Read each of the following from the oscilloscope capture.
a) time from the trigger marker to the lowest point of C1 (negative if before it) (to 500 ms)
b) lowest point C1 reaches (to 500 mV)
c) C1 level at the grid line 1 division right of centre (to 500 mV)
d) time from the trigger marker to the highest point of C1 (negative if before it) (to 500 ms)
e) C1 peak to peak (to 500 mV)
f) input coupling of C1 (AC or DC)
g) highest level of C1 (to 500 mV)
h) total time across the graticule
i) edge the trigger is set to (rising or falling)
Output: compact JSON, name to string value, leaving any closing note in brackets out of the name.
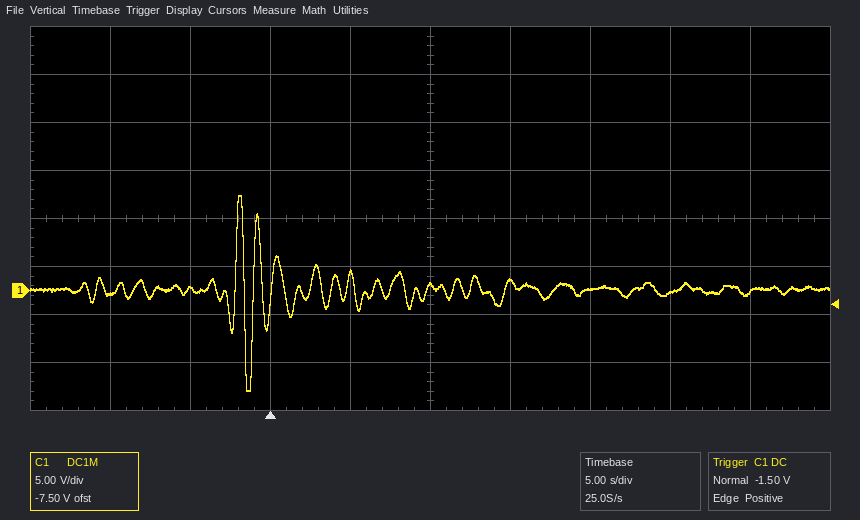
{"time from the trigger marker to the lowest point of C1 (negative if before it)": "-1.5 s", "lowest point C1 reaches": "-10.5 V", "C1 level at the grid line 1 division right of centre": "1.0 V", "time from the trigger marker to the highest point of C1 (negative if before it)": "-2.0 s", "C1 peak to peak": "20.5 V", "input coupling of C1": "DC", "highest level of C1": "10.0 V", "total time across the graticule": "50 s", "edge the trigger is set to": "rising"}
